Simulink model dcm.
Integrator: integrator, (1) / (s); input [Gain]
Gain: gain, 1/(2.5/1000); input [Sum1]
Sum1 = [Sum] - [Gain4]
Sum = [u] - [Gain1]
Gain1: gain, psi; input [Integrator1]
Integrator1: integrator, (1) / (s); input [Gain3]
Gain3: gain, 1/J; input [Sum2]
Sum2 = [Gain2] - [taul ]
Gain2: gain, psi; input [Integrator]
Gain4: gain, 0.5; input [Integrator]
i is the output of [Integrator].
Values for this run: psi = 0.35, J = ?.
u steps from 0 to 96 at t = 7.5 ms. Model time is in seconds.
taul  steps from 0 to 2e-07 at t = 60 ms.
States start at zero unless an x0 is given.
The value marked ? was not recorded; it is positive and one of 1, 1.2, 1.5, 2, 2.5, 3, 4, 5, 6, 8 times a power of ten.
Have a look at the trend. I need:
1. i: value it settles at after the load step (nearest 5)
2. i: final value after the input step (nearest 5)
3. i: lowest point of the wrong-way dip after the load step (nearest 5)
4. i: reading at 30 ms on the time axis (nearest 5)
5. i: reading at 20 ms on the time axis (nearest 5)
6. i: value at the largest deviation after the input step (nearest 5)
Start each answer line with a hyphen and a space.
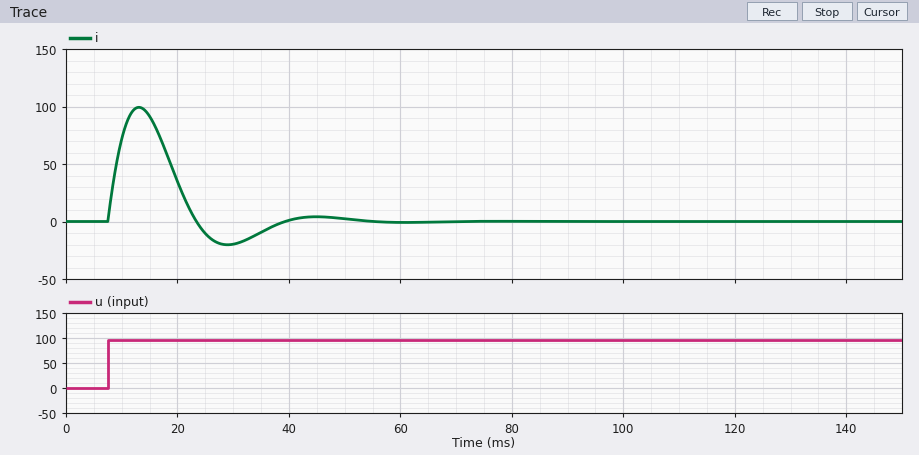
- 0
- 0
- 0
- -20
- 35
- 100
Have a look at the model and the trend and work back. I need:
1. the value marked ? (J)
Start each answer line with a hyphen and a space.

- 0.001
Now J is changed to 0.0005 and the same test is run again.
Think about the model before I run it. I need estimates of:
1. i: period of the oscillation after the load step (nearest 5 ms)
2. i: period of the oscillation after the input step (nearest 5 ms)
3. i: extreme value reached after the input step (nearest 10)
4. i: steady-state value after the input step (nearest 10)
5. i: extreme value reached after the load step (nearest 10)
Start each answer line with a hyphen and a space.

- 20 ms
- 20 ms
- 80
- 0
- 0
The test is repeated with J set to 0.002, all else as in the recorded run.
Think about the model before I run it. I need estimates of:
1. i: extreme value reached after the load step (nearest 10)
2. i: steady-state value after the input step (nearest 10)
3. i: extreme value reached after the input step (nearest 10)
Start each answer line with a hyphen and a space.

- 0
- 0
- 120
